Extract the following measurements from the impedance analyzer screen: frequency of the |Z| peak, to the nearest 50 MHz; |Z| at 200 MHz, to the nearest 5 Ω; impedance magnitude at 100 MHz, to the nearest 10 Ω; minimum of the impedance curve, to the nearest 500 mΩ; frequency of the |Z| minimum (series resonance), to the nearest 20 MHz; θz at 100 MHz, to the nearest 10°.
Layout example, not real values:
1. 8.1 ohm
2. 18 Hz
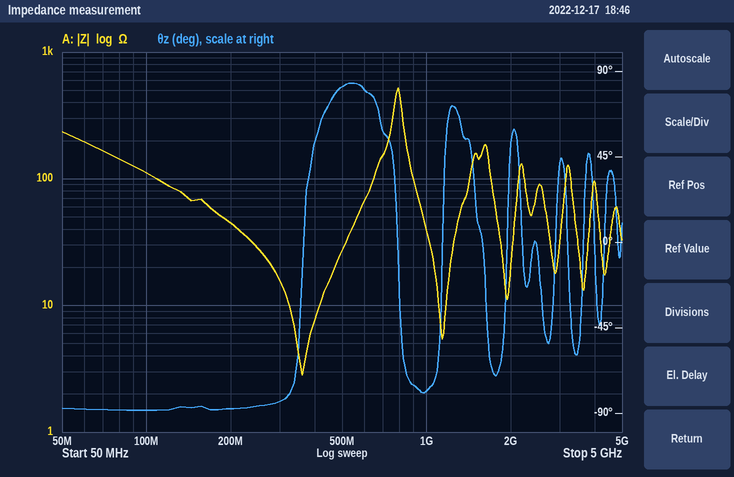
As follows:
1. 800 MHz
2. 45 Ω
3. 110 Ω
4. 3.0 Ω
5. 360 MHz
6. -90°
